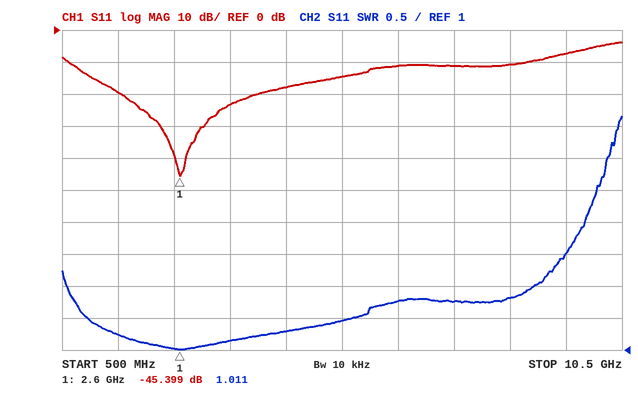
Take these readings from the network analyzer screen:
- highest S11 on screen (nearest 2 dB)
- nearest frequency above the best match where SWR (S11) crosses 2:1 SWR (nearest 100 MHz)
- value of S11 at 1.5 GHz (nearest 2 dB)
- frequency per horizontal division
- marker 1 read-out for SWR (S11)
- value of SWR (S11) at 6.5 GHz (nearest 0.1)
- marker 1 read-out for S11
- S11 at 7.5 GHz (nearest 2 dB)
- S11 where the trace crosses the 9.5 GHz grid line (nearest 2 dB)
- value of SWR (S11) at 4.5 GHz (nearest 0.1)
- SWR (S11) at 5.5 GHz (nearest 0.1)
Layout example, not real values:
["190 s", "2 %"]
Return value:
["-4 dB", "8.9 GHz", "-20 dB", "1 GHz", "1.011", "1.8", "-45.399 dB", "-12 dB", "-8 dB", "1.3", "1.5"]
